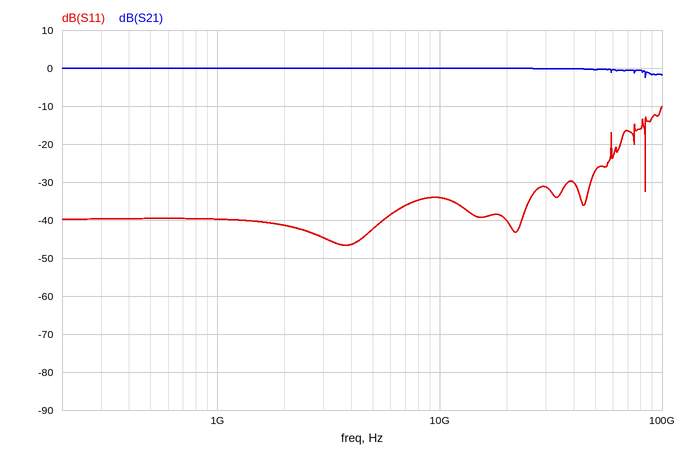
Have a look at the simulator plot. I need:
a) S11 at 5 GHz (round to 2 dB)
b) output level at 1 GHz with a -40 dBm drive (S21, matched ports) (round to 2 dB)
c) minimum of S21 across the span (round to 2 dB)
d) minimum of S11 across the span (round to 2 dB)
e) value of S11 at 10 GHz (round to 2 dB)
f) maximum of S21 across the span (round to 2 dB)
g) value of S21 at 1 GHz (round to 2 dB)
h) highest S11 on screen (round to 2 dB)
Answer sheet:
-42 dB
-40 dBm
-2 dB
-46 dB
-34 dB
0 dB
0 dB
-10 dB
